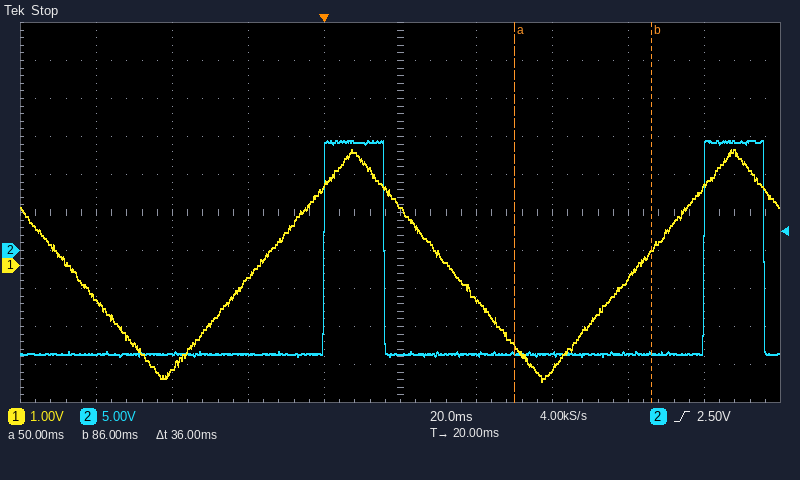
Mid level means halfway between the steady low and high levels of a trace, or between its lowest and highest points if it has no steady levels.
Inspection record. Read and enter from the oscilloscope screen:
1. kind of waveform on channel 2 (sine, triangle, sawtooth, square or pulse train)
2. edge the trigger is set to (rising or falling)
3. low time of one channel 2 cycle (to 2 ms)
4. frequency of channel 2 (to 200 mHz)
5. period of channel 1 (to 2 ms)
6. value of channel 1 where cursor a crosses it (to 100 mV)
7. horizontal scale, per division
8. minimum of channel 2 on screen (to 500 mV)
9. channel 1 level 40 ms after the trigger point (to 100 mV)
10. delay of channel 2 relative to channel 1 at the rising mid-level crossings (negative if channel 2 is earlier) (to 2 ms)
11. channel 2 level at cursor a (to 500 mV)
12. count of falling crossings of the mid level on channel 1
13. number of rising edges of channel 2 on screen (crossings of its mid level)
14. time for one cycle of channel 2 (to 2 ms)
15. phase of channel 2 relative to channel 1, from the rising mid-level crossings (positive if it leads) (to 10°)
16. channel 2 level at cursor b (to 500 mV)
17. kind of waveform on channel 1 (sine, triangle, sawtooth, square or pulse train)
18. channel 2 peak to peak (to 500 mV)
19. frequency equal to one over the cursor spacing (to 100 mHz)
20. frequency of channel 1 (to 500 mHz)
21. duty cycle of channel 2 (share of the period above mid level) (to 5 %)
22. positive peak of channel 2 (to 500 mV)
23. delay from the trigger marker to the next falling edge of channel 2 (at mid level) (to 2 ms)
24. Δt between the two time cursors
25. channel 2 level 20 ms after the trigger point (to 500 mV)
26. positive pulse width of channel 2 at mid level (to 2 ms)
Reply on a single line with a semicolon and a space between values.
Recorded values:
pulse train; rising; 84 ms; 10.0 Hz; 100 ms; -2.1 V; 20 ms; -14.0 V; -900 mV; +18 ms; -13.5 V; 2; 2; 100 ms; -60°; -13.5 V; triangle; 28.5 V; 27.8 Hz; 10.0 Hz; 15 %; 14.5 V; 16 ms; 36 ms; -13.5 V; 16 ms
